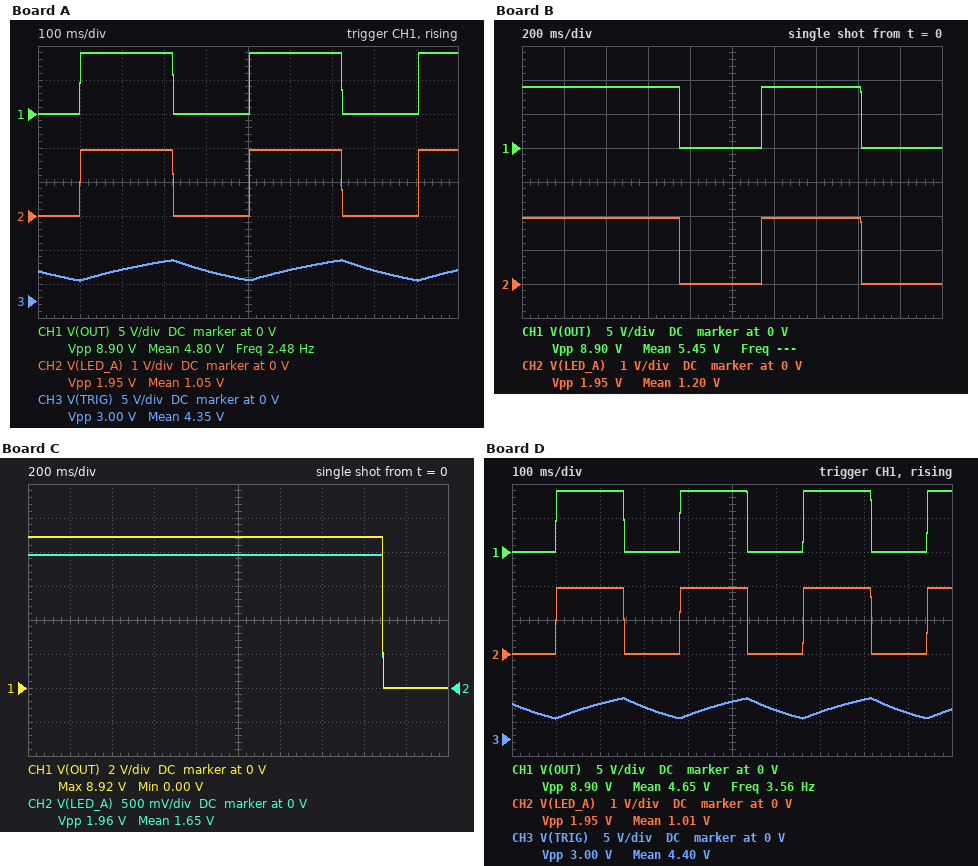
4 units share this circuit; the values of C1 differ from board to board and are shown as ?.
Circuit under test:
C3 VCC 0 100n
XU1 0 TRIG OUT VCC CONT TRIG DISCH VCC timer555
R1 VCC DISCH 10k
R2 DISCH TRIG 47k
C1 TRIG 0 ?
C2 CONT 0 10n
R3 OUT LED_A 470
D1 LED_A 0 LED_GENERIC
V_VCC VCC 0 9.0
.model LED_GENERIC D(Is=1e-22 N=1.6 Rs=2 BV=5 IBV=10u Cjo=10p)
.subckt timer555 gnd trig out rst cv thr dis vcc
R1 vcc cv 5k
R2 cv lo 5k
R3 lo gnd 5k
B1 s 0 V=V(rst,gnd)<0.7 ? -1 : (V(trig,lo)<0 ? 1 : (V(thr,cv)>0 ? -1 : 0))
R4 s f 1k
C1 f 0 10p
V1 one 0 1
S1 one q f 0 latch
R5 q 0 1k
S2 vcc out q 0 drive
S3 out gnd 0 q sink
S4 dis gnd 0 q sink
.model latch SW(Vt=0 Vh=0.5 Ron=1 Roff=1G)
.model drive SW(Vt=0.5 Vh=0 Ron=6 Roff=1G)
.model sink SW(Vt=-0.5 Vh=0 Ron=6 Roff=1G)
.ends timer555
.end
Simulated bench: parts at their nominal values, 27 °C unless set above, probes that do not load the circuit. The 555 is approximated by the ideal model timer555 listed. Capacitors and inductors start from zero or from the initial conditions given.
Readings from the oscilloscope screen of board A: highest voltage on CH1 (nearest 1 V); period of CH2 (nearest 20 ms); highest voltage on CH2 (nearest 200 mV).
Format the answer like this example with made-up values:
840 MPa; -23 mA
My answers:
9 V; 400 ms; 2.0 V
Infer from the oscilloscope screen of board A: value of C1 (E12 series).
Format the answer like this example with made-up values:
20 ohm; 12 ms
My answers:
5.6 µF
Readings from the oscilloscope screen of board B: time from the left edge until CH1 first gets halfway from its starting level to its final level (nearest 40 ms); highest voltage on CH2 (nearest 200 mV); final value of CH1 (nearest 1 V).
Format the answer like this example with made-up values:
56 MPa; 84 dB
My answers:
760 ms; 2.0 V; 0 V
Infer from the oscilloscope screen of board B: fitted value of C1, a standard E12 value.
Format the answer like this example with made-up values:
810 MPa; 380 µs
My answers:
12 µF
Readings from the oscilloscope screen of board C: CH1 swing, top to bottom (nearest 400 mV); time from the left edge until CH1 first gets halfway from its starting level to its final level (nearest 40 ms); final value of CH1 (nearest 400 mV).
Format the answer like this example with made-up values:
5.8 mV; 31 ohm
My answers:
8.8 V; 1.68 s; 0 V
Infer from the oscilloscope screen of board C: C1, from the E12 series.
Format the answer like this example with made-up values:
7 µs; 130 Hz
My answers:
27 µF
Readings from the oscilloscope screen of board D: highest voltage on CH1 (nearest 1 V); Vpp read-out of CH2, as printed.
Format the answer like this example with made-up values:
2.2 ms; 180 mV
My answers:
9 V; 1.95 V
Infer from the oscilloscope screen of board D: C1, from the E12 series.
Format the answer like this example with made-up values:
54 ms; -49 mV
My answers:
3.9 µF
